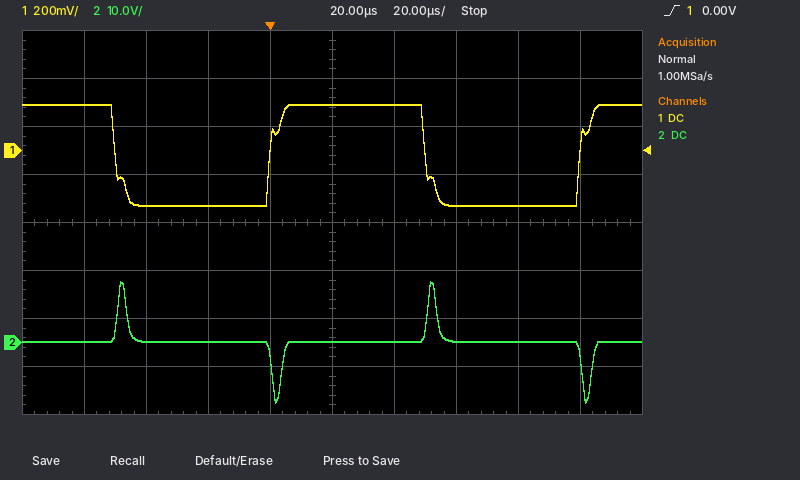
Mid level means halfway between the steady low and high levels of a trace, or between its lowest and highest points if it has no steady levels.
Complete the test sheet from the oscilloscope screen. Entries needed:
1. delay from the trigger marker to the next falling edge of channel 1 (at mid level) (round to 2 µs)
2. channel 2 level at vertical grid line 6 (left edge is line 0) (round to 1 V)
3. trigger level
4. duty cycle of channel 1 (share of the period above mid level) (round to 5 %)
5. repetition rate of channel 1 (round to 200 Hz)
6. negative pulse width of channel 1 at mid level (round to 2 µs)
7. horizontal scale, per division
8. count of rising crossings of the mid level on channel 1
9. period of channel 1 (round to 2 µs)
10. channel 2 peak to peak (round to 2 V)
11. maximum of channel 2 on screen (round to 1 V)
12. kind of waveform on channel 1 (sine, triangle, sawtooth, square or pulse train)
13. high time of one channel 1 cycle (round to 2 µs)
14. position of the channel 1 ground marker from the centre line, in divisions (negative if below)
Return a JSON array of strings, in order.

["50 µs", "0 V", "0.00 V", "50 %", "10.0 kHz", "50 µs", "20 µs", "2", "100 µs", "26 V", "13 V", "square", "50 µs", "+1.5 div"]
